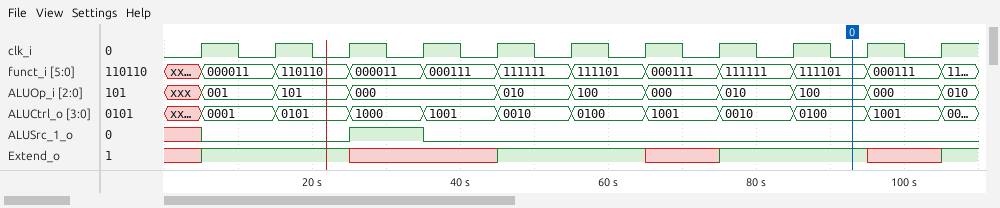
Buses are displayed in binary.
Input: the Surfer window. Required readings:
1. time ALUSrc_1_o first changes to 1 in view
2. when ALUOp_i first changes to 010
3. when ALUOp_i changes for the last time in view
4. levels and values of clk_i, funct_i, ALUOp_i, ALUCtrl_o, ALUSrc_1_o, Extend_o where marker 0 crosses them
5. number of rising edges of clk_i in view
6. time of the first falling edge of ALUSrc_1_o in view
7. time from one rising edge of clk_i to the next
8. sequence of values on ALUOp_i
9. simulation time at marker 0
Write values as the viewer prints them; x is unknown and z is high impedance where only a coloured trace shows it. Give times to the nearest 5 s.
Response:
25 s
45 s
105 s
clk_i=0, funct_i=111101, ALUOp_i=100, ALUCtrl_o=0100, ALUSrc_1_o=0, Extend_o=1
11
35 s
10 s
xxx, 001, 101, 000, 010, 100, 000, 010, 100, 000, 010
95 s
